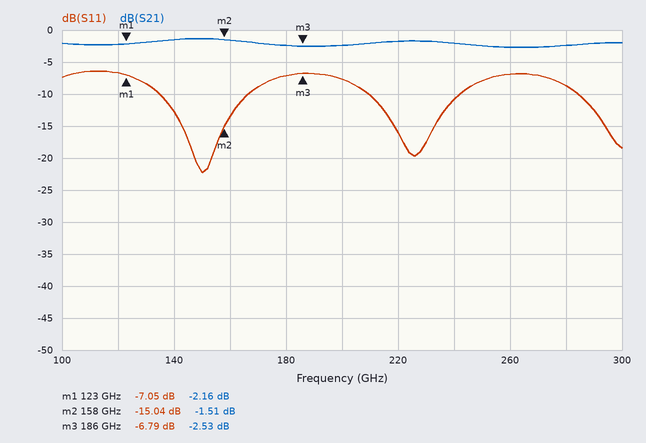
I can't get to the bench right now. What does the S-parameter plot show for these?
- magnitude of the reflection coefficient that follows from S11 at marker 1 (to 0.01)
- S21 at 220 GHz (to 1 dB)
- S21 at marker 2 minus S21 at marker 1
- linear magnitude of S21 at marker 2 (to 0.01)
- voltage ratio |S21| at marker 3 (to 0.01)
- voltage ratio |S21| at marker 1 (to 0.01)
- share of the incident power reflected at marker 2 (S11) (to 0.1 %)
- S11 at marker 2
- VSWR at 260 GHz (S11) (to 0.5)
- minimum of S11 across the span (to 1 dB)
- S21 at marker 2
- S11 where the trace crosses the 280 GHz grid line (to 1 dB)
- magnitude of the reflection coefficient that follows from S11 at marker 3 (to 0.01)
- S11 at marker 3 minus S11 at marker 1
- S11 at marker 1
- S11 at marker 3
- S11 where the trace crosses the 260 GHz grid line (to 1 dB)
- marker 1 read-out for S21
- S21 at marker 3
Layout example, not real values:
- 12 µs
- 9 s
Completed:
- 0.44
- -2 dB
- 0.65 dB
- 0.84
- 0.75
- 0.78
- 3.1 %
- -15.04 dB
- 2.5
- -22 dB
- -1.51 dB
- -9 dB
- 0.46
- 0.26 dB
- -7.05 dB
- -6.79 dB
- -7 dB
- -2.16 dB
- -2.53 dB
